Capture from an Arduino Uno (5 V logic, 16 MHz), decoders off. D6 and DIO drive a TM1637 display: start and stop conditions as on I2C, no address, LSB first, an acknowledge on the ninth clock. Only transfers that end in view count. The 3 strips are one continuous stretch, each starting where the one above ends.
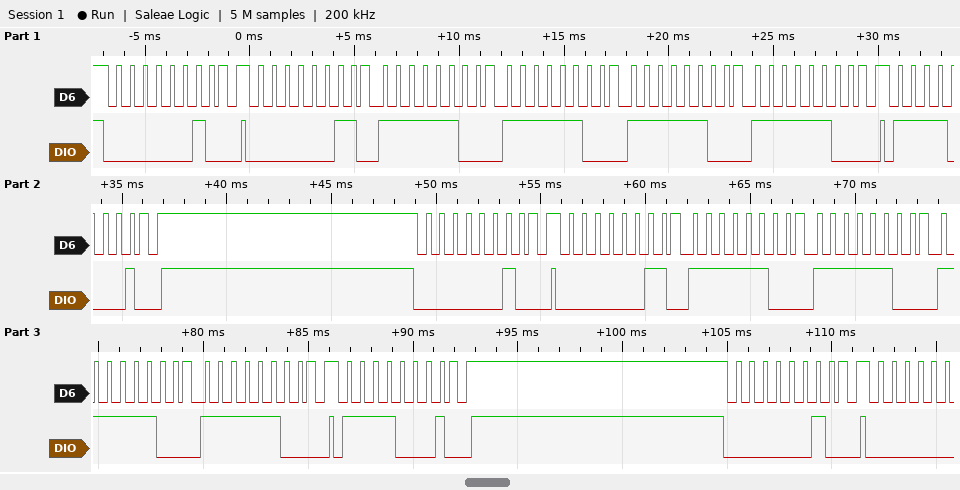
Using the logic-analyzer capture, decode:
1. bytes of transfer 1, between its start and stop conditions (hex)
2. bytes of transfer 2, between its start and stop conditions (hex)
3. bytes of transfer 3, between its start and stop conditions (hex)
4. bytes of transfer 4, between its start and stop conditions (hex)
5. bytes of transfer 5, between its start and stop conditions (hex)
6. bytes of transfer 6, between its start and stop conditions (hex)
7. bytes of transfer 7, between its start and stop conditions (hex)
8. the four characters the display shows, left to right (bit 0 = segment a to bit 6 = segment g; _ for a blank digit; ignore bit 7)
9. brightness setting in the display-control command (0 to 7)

40
C0 3F 3F 3F 3F
8F
40
C0 3F 3F 3F 3F
8F
40
0000
7
